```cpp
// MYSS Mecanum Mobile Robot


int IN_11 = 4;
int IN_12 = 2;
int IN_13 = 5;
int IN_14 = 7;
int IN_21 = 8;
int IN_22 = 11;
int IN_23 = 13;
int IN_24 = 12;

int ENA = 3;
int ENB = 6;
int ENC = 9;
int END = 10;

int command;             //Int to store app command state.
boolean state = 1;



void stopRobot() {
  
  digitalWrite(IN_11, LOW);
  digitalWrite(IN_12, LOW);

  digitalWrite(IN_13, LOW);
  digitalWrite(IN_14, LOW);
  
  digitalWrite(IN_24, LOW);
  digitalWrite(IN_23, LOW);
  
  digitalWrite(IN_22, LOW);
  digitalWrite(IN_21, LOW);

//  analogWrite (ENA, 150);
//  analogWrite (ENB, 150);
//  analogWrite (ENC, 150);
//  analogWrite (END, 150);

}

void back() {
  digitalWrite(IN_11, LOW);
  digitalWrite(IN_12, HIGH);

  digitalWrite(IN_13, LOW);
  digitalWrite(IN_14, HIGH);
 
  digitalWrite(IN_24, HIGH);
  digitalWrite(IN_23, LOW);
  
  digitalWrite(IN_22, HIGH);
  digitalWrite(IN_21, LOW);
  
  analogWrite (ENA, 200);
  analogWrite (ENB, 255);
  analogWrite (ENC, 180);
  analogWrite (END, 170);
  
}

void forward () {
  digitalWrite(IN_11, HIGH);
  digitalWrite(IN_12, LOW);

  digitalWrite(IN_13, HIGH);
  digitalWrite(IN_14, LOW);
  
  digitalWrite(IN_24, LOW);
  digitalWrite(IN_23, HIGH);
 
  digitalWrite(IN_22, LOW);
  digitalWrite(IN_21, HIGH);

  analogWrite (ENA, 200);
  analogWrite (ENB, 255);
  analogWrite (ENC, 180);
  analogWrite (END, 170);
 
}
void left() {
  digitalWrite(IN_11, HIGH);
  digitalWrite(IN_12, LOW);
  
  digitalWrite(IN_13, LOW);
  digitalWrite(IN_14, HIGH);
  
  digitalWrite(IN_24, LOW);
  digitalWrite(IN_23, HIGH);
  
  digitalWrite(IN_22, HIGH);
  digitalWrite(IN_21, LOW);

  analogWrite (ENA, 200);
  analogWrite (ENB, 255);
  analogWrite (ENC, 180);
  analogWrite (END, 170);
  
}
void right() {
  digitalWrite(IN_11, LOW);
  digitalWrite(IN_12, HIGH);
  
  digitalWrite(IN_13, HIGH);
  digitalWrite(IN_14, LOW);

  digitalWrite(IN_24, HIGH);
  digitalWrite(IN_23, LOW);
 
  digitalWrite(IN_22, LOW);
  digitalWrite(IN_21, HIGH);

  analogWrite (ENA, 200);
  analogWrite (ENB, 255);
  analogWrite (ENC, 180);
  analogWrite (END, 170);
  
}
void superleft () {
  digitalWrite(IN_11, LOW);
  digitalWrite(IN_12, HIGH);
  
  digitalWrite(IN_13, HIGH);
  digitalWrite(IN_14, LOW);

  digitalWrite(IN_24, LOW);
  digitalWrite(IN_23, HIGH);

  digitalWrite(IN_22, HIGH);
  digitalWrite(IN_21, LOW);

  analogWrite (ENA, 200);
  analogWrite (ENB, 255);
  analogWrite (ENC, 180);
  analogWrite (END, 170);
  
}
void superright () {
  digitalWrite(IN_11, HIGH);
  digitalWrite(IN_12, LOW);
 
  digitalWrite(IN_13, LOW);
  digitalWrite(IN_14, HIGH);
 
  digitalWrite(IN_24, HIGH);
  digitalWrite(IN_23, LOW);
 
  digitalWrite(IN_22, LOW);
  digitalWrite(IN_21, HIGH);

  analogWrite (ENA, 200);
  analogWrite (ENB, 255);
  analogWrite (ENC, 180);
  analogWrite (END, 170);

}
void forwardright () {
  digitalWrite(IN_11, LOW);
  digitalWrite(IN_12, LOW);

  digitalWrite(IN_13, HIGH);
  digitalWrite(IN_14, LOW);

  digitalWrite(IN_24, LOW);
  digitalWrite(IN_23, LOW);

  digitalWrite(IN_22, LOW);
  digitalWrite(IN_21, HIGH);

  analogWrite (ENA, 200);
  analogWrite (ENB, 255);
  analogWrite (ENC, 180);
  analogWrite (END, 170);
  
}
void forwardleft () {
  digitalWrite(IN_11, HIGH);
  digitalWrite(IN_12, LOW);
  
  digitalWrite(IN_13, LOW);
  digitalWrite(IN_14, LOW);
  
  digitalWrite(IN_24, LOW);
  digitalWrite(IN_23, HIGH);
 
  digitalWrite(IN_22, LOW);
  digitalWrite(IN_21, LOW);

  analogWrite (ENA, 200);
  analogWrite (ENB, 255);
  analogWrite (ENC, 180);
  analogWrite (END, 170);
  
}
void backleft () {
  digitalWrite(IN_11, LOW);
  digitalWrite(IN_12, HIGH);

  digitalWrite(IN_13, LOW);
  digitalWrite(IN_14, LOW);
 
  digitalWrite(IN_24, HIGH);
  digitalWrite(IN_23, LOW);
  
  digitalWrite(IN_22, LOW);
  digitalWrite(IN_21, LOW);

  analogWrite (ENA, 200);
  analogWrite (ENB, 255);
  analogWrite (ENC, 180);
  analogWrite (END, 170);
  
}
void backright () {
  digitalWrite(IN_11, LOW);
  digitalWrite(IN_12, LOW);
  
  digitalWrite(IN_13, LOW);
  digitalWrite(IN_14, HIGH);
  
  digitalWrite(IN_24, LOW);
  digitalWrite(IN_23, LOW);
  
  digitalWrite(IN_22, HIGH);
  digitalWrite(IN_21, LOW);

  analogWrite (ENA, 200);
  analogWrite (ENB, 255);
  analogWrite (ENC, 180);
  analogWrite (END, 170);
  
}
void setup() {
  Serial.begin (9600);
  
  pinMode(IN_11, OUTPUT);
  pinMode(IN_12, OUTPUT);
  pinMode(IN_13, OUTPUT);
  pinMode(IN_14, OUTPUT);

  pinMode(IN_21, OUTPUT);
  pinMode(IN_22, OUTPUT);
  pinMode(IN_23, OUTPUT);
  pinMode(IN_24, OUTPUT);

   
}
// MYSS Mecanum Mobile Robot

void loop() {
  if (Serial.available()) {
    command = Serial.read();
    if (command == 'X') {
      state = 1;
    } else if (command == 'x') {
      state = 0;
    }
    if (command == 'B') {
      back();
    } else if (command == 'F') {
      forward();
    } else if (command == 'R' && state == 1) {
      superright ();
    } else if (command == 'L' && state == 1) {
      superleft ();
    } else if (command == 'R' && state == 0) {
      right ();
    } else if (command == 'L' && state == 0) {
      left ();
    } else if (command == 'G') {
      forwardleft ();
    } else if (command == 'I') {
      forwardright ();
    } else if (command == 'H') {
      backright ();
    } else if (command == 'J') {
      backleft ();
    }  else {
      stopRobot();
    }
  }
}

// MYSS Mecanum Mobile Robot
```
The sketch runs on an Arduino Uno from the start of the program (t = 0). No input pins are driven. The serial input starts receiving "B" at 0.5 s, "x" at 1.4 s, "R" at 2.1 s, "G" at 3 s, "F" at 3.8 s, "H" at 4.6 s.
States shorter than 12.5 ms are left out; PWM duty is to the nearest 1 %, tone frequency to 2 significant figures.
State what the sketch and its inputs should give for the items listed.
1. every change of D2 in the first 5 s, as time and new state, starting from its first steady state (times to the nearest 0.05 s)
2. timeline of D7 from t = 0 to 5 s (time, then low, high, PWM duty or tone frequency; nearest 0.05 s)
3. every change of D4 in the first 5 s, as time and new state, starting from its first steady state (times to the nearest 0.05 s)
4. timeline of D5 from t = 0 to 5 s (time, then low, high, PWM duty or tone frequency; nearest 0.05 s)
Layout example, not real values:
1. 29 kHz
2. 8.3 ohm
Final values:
1. 0 s low; 0.5 s high; 1.4 s low; 2.1 s high; 3 s low
2. 0 s low; 0.5 s high; 1.4 s low; 4.6 s high
3. 0 s low; 3 s high; 4.6 s low
4. 0 s low; 2.1 s high; 3 s low; 3.8 s high; 4.6 s low
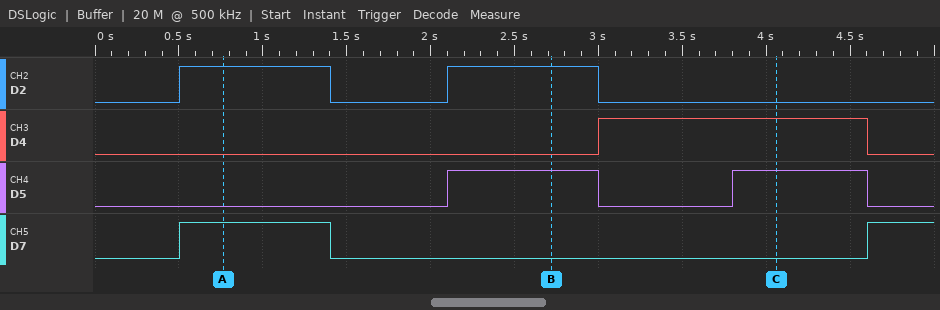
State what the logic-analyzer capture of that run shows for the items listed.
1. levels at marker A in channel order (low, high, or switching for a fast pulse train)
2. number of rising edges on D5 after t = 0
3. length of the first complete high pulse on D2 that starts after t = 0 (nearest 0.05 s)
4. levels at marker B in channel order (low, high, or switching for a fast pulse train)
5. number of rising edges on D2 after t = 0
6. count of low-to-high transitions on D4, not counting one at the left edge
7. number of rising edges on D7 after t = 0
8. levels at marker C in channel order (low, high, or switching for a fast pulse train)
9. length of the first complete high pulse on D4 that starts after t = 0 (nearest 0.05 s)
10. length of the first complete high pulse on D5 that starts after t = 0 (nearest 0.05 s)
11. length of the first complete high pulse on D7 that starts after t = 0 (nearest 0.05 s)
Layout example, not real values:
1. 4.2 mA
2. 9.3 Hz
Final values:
1. D2 high, D4 low, D5 low, D7 high
2. 2
3. 0.90 s
4. D2 high, D4 low, D5 high, D7 low
5. 2
6. 1
7. 2
8. D2 low, D4 high, D5 high, D7 low
9. 1.60 s
10. 0.90 s
11. 0.90 s
